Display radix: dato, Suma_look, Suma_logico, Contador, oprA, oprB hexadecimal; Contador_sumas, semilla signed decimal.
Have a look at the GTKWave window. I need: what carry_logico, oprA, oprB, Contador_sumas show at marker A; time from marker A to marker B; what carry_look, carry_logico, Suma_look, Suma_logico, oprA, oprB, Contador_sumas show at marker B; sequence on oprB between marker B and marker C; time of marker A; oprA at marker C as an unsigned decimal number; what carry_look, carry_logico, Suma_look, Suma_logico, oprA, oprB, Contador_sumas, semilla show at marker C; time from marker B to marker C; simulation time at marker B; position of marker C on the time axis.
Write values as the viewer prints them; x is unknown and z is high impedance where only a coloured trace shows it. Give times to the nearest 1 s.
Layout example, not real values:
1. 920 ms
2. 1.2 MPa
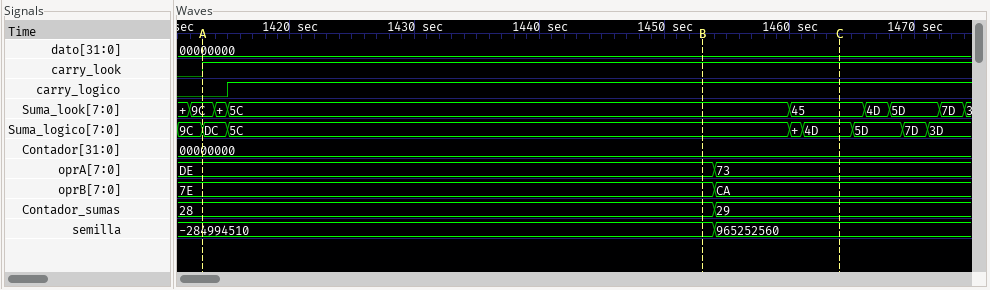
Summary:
1. carry_logico=0, oprA=DE, oprB=7E, Contador_sumas=28
2. 40 s
3. carry_look=1, carry_logico=1, Suma_look=5C, Suma_logico=5C, oprA=DE, oprB=7E, Contador_sumas=28
4. 7E, CA
5. 1413 s
6. 115
7. carry_look=1, carry_logico=1, Suma_look=45, Suma_logico=4D, oprA=73, oprB=CA, Contador_sumas=29, semilla=965252560
8. 11 s
9. 1453 s
10. 1464 s
